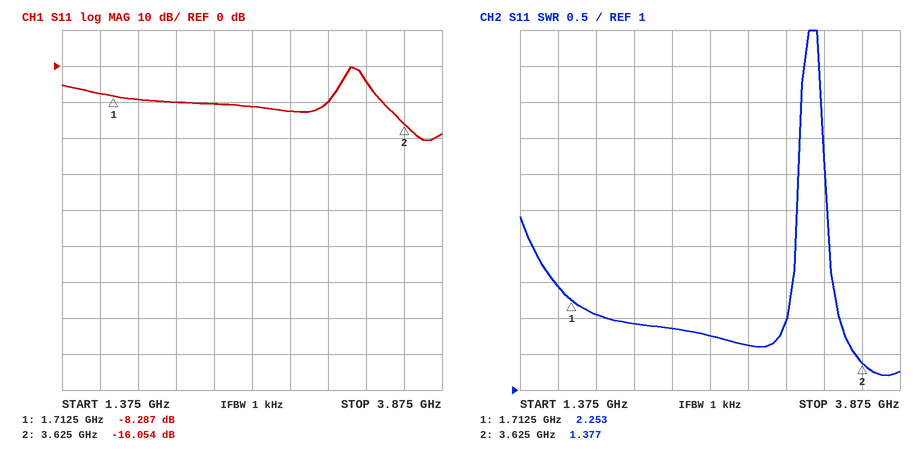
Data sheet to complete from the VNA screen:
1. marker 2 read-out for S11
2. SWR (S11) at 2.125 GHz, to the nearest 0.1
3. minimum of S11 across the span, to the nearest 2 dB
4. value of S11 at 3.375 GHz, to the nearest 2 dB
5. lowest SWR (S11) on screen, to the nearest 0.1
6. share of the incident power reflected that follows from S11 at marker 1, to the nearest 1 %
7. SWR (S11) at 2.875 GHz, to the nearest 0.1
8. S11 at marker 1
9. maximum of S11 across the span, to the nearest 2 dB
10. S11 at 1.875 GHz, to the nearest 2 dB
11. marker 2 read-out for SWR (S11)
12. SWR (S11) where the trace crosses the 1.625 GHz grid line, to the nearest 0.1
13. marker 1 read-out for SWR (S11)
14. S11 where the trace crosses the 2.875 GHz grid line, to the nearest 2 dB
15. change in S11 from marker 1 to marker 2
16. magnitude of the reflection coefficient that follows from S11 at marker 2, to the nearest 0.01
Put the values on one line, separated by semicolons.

-16.054 dB; 1.9; -20 dB; -4 dB; 1.2; 15 %; 1.6; -8.287 dB; 0 dB; -10 dB; 1.377; 2.4; 2.253; -12 dB; -7.767 dB; 0.16
